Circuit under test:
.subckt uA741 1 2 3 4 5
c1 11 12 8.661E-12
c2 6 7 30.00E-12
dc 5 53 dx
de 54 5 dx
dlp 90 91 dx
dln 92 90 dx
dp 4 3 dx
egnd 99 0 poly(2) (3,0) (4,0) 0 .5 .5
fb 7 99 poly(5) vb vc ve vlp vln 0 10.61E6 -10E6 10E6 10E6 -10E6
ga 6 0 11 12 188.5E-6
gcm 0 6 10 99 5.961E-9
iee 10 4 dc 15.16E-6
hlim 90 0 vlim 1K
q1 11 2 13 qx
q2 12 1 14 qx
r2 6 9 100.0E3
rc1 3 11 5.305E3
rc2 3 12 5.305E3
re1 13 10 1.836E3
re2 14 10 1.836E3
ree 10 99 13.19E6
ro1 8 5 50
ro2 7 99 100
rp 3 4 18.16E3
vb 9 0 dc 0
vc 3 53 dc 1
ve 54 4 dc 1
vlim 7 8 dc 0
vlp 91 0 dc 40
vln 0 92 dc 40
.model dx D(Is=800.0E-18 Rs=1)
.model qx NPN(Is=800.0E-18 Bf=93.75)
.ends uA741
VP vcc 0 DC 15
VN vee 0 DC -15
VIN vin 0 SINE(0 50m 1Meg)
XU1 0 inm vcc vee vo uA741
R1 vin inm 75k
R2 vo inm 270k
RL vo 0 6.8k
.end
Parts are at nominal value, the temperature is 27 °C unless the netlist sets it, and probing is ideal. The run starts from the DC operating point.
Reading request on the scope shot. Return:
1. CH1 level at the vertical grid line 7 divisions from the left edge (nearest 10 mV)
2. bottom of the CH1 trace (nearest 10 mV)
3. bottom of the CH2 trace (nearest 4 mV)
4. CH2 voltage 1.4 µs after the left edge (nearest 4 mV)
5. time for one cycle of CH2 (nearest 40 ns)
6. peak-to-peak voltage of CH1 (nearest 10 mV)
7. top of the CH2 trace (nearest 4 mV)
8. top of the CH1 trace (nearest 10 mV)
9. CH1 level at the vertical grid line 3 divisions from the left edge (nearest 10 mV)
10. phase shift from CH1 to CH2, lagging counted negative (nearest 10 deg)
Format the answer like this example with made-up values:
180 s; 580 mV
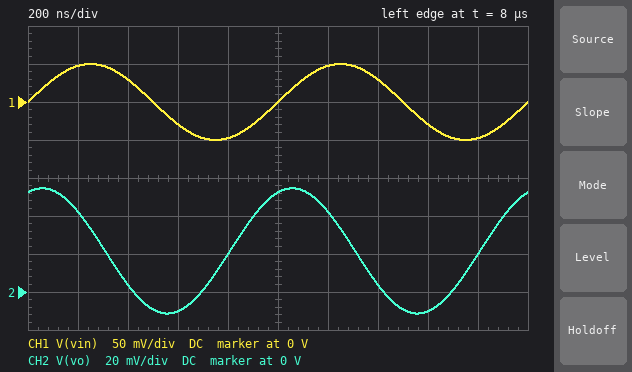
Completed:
30 mV; -50 mV; -12 mV; 4 mV; 1.00 µs; 100 mV; 56 mV; 50 mV; -30 mV; 70 deg
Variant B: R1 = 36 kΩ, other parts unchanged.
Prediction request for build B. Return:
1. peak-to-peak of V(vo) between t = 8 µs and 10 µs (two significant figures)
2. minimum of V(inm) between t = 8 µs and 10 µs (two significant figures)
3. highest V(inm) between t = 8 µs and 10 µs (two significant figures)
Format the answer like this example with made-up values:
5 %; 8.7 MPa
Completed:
73 mV; -45 mV; 45 mV
